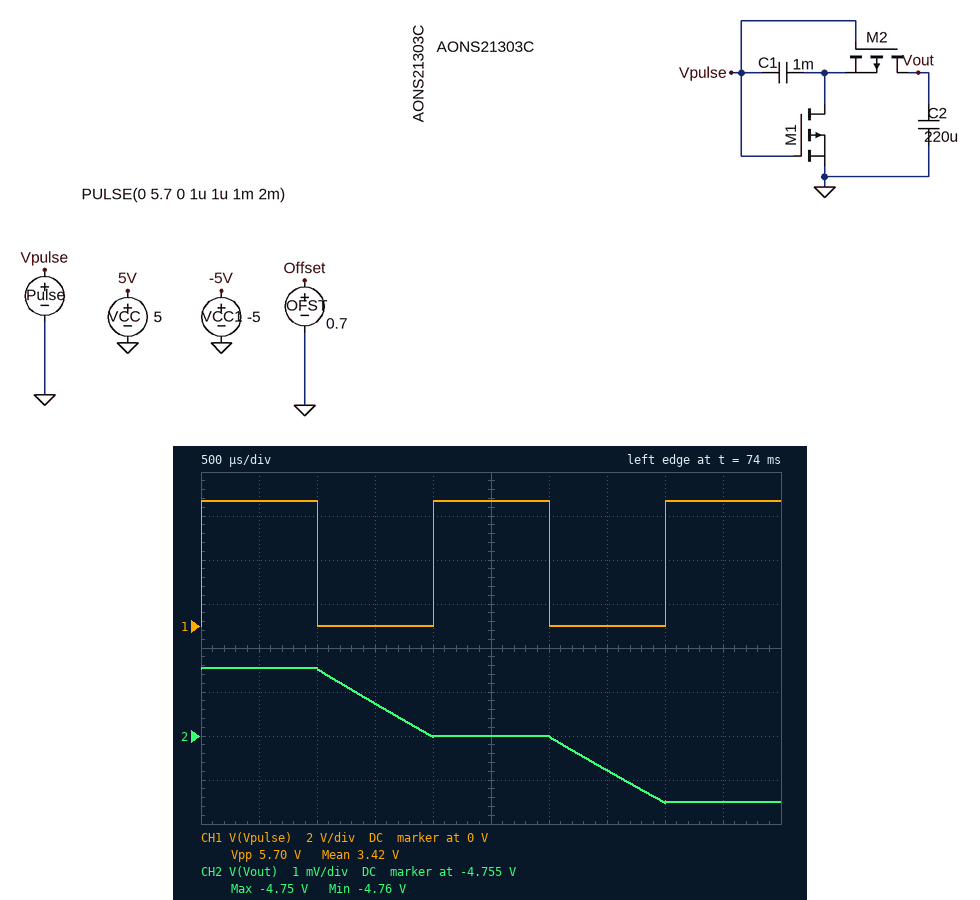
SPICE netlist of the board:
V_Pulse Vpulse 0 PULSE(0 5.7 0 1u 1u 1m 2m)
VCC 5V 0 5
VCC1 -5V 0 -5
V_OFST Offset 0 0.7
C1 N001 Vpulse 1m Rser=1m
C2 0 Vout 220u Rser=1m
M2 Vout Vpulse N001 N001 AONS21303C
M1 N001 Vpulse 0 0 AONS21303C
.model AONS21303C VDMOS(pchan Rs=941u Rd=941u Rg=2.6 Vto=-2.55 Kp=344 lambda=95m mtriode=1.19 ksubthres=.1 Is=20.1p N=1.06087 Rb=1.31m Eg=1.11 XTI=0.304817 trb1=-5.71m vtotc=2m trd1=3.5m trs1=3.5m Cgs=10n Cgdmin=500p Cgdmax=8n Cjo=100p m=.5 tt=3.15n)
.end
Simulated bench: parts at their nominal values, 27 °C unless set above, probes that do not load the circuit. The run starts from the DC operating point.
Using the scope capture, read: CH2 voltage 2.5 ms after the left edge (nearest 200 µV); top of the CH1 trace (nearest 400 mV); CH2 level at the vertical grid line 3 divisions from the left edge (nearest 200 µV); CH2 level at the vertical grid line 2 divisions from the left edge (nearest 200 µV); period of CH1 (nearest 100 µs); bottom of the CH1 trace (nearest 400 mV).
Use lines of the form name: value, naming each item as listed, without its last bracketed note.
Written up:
CH2 voltage 2.5 ms after the left edge: -4.7550 V
top of the CH1 trace: 5.6 V
CH2 level at the vertical grid line 3 divisions from the left edge: -4.7542 V
CH2 level at the vertical grid line 2 divisions from the left edge: -4.7534 V
period of CH1: 2.0 ms
bottom of the CH1 trace: 0 V
